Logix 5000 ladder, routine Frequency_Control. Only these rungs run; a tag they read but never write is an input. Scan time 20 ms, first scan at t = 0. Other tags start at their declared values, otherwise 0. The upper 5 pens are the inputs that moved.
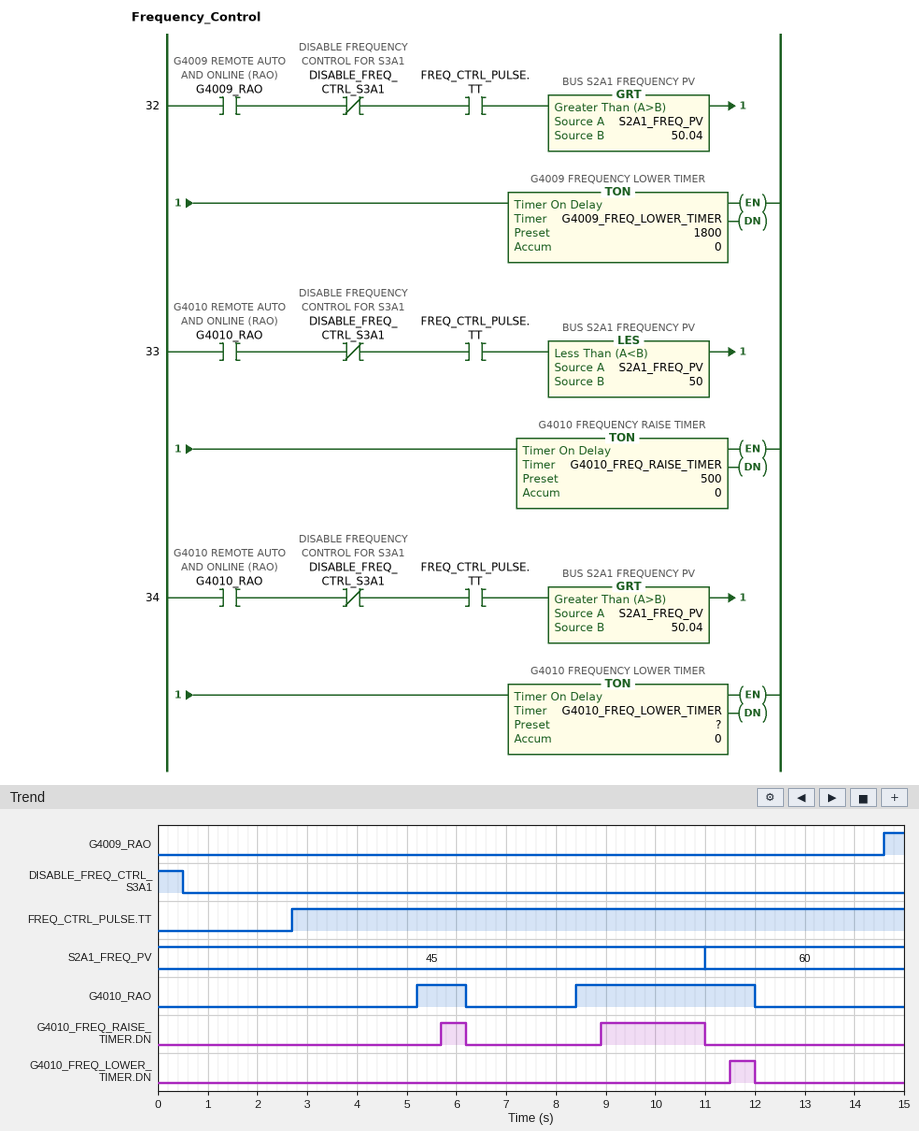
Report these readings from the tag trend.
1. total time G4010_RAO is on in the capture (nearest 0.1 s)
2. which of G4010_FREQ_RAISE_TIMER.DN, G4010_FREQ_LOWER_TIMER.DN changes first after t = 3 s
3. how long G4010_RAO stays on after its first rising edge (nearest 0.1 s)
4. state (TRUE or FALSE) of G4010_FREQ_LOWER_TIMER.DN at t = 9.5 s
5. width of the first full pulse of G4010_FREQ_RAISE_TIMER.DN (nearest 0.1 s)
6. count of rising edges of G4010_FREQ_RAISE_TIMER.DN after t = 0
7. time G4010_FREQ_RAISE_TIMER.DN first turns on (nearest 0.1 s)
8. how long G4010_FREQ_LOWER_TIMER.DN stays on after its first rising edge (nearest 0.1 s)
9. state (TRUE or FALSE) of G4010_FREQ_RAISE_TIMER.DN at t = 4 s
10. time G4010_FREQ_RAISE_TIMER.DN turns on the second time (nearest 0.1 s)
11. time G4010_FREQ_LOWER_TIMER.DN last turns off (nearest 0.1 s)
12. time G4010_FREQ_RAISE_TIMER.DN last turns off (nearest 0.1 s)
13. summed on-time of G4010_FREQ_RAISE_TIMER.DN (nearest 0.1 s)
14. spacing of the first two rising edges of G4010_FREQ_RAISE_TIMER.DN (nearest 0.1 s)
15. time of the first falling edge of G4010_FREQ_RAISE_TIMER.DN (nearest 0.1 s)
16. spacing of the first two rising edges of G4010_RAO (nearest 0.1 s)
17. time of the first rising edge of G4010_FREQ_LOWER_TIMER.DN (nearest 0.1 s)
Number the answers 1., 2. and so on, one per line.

1. 4.6 s
2. G4010_FREQ_RAISE_TIMER.DN
3. 1.0 s
4. FALSE
5. 0.5 s
6. 2
7. 5.7 s
8. 0.5 s
9. FALSE
10. 8.9 s
11. 12.0 s
12. 11.0 s
13. 2.6 s
14. 3.2 s
15. 6.2 s
16. 3.2 s
17. 11.5 s
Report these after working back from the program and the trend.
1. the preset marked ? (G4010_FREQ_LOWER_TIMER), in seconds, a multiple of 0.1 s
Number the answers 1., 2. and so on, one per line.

1. 0.5 s
